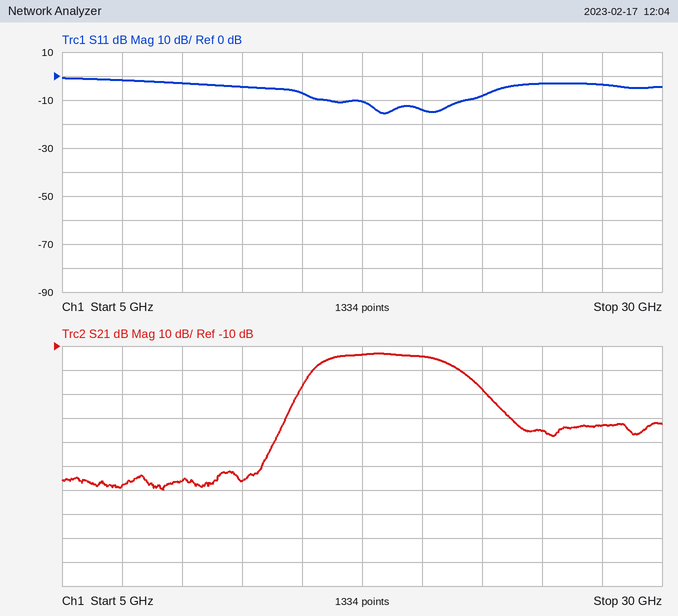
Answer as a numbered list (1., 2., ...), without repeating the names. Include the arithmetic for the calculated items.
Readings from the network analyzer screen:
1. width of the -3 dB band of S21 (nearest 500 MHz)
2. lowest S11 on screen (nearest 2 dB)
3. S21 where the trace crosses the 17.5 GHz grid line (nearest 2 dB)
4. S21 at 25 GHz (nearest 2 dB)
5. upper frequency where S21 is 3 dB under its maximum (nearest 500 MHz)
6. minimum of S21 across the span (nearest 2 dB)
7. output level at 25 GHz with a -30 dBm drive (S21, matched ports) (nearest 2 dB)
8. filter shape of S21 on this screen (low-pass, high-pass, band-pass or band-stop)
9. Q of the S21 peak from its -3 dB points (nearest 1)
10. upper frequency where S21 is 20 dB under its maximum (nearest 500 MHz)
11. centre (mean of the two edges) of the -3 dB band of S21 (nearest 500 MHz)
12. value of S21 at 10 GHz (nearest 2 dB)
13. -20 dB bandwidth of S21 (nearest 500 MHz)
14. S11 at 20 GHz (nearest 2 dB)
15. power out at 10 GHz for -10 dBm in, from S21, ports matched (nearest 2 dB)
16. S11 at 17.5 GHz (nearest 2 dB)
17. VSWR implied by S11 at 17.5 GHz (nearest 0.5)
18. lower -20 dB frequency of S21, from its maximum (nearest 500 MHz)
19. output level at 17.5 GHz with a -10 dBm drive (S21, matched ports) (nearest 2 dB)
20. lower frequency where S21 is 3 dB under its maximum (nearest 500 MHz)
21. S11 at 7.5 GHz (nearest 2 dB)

1. 21.0 GHz − 16.0 GHz = 5.0 GHz
2. -16 dB
3. -14 dB
4. -46 dB
5. 21.0 GHz
6. -70 dB
7. -30 dBm + (-46 dB) = -76 dBm
8. band-pass
9. 18.5 GHz / 5 GHz ≈ 4
10. 23.0 GHz
11. 18.5 GHz
12. -66 dB
13. 23.0 GHz − 14.5 GHz = 8.5 GHz
14. -14 dB
15. -10 dBm + (-66 dB) = -76 dBm
16. -10 dB
17. |Γ| = 10^(-10/20) = 0.3162; VSWR = (1 + 0.3162)/(1 − 0.3162) ≈ 1.92, so 2.0 to the nearest 0.5
18. 14.5 GHz
19. -10 dBm + (-14 dB) = -24 dBm
20. 16.0 GHz
21. -2 dB
